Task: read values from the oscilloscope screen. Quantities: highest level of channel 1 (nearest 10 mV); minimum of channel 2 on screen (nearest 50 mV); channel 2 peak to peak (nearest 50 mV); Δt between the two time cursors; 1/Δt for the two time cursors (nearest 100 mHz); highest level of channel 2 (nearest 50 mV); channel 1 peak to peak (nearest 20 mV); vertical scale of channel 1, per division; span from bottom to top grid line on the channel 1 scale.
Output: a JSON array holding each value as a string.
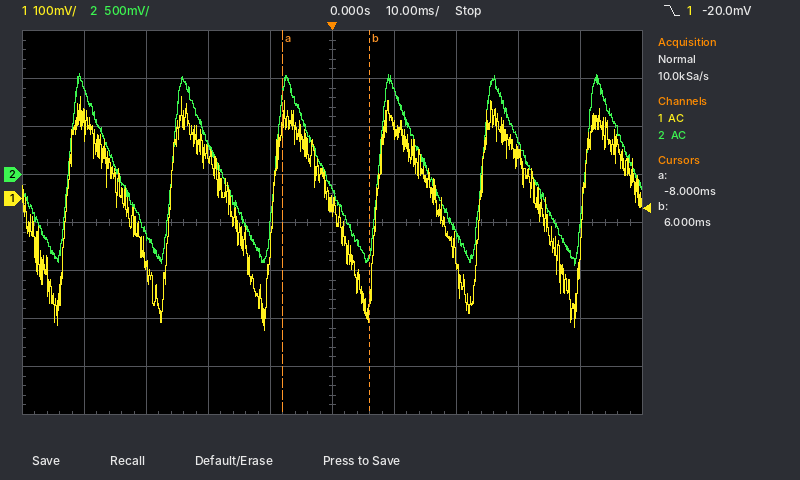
["210 mV", "-950 mV", "2.00 V", "14 ms", "71.4 Hz", "1.05 V", "480 mV", "100 mV", "800 mV"]
